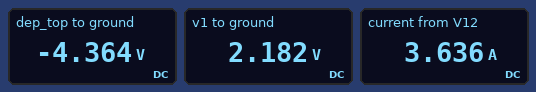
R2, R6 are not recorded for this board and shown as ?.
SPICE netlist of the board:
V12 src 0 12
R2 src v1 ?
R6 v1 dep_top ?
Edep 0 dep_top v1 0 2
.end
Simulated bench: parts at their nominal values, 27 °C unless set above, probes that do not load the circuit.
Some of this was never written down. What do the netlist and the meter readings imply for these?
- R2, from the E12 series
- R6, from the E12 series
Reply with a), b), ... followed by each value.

a) 2.7 Ω
b) 1.8 Ω
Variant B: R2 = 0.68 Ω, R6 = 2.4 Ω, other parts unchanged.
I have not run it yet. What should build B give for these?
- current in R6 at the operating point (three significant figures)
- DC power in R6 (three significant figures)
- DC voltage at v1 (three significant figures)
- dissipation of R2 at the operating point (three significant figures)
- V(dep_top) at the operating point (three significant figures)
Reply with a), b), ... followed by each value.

a) 8.11 A
b) 158 W
c) 6.49 V
d) 44.7 W
e) -13.0 V
